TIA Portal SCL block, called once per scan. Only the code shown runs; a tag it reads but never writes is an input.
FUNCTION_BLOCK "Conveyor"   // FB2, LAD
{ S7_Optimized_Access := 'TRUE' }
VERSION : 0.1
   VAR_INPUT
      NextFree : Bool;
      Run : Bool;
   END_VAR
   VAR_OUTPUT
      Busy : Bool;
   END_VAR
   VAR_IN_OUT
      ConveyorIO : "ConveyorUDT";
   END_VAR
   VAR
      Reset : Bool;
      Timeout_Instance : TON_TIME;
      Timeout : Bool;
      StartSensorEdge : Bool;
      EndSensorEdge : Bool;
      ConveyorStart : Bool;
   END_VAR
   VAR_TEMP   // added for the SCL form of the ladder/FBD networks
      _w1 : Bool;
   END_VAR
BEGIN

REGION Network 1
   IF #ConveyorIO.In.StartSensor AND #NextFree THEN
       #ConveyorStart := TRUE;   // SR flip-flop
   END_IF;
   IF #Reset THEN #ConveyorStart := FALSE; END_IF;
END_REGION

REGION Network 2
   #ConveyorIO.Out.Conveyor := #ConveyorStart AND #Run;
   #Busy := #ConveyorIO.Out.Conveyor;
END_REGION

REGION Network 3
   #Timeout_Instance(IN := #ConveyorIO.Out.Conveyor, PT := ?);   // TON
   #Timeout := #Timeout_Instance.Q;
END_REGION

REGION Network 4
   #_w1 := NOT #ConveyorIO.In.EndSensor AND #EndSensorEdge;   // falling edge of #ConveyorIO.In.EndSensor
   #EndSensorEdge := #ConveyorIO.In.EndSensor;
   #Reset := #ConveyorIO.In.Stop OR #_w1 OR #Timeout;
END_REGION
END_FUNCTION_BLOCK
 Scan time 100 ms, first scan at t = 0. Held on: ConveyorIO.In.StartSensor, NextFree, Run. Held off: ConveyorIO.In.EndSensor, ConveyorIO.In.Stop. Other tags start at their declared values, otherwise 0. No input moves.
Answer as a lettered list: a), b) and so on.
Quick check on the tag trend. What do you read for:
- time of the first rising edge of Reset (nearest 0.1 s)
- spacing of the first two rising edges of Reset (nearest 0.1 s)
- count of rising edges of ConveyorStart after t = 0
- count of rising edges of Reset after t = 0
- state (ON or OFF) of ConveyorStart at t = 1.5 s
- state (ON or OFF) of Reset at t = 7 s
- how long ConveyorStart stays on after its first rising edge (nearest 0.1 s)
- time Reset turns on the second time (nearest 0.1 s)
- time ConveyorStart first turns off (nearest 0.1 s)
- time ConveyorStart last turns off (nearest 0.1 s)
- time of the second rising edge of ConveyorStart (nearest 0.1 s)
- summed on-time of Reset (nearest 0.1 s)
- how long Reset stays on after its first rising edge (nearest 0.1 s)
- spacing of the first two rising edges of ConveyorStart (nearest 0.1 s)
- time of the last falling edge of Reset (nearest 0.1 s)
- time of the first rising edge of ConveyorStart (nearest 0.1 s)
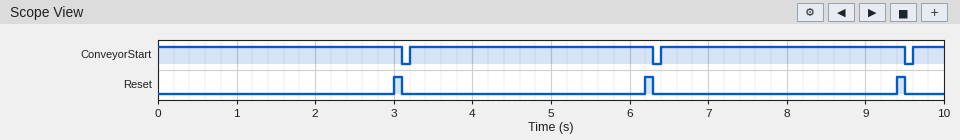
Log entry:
a) 3.0 s
b) 3.2 s
c) 3
d) 3
e) ON
f) OFF
g) 3.1 s
h) 6.2 s
i) 3.1 s
j) 9.5 s
k) 6.4 s
l) 0.3 s
m) 0.1 s
n) 3.2 s
o) 9.5 s
p) 3.2 s
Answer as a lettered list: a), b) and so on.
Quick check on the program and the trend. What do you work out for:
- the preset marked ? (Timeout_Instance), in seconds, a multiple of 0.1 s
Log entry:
a) 3.0 s
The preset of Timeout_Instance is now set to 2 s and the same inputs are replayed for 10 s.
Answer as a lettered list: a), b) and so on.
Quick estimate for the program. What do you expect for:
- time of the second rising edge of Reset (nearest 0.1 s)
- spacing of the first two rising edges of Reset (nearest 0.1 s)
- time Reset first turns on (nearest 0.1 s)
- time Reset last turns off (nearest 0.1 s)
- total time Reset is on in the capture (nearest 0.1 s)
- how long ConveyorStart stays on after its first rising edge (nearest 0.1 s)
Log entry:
a) 4.2 s
b) 2.2 s
c) 2.0 s
d) 8.7 s
e) 0.4 s
f) 2.1 s
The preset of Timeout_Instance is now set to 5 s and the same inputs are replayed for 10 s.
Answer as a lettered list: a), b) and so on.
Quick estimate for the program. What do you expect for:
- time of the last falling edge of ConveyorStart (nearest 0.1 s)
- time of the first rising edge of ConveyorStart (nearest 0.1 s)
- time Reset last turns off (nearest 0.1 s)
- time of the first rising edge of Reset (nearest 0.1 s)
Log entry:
a) 5.1 s
b) 5.2 s
c) 5.1 s
d) 5.0 s
